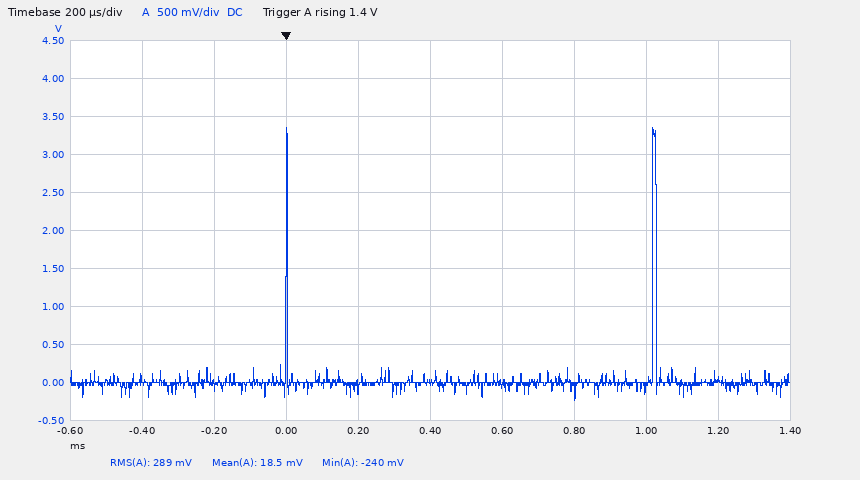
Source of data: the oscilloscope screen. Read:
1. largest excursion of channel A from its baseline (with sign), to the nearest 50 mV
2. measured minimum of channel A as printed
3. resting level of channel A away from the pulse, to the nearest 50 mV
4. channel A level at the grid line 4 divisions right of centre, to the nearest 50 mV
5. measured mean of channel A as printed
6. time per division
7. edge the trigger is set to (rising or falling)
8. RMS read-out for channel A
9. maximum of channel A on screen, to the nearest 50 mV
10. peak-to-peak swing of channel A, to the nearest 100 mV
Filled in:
+3.35 V
-240 mV
0 mV
50 mV
18.5 mV
200 µs
rising
289 mV
3.35 V
3.60 V
